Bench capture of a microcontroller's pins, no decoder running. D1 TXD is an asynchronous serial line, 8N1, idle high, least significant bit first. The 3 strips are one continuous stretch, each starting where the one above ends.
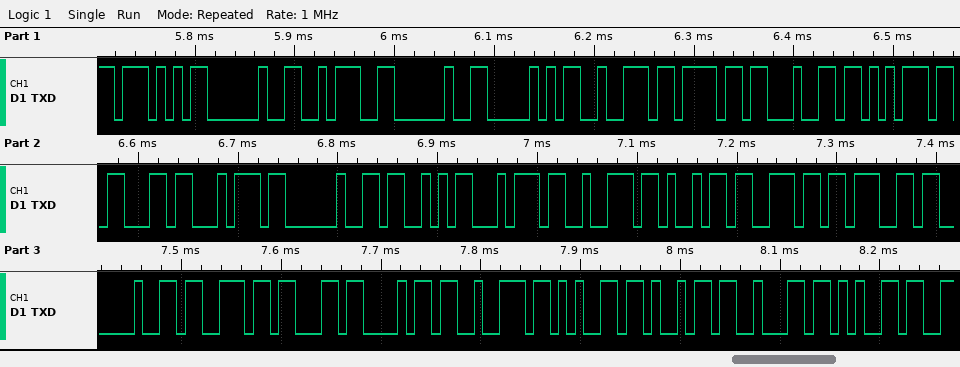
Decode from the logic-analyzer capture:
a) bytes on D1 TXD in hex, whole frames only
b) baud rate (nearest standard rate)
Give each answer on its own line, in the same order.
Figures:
57 20 3A 20 50 72 6F 64 75 63 74 20 53 74 72 69 6E 67 20 73 63 68 72 65 69 62 65
115200 baud
